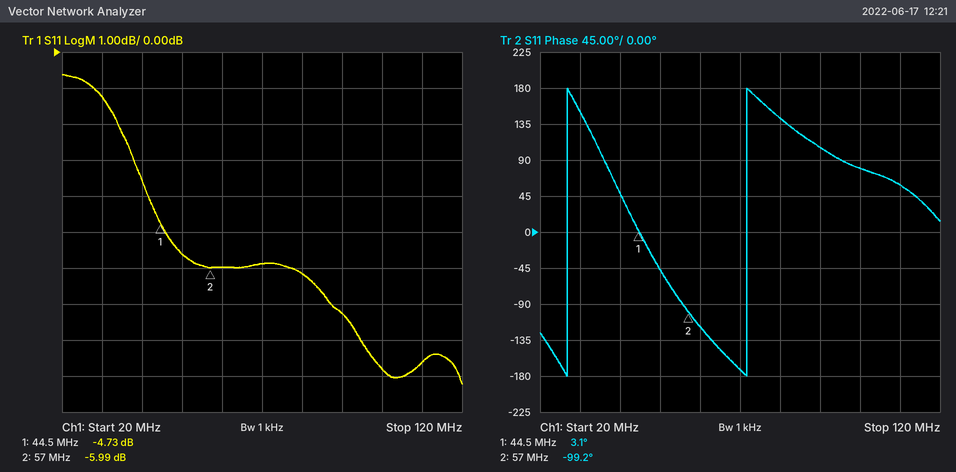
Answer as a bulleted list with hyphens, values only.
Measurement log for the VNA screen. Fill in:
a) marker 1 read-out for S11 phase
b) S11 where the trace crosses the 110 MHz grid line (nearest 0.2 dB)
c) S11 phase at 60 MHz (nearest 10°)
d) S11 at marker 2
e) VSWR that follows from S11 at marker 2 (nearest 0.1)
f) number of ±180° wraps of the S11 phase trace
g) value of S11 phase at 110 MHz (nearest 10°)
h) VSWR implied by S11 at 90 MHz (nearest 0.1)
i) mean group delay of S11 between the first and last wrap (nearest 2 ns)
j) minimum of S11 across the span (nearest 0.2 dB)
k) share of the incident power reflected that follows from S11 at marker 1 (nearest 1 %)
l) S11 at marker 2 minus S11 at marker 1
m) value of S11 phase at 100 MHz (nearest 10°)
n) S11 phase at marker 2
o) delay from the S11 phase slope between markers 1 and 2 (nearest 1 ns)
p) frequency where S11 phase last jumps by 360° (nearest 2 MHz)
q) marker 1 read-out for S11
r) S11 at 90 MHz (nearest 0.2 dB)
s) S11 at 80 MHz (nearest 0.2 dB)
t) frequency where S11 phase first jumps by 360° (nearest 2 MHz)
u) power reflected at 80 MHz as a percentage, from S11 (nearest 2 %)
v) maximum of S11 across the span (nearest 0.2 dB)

- 3.1°
- -8.6 dB
- -120°
- -5.99 dB
- 3.0
- 2
- 60°
- 2.5
- 22 ns
- -9.2 dB
- 34 %
- -1.26 dB
- 80°
- -99.2°
- 23 ns
- 72 MHz
- -4.73 dB
- -7.2 dB
- -6.2 dB
- 26 MHz
- 24 %
- -0.6 dB
